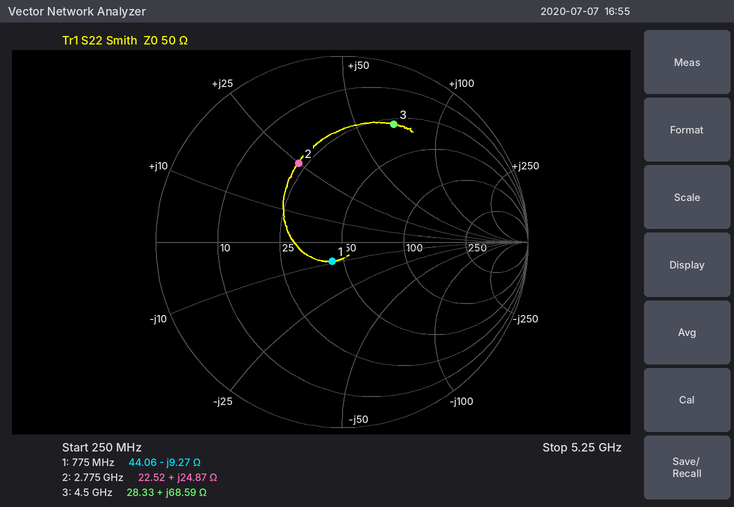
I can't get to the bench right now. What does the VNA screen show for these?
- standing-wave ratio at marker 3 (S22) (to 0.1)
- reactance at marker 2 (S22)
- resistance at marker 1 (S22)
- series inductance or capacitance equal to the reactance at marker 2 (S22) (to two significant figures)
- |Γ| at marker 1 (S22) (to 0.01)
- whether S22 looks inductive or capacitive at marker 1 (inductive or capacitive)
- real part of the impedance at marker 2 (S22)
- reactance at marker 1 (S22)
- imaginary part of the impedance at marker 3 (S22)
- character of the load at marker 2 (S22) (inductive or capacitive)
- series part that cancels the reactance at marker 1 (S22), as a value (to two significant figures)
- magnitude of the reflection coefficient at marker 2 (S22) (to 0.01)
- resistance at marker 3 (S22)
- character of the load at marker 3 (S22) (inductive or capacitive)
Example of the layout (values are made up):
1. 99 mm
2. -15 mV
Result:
1. 5.5
2. +24.87 Ω
3. 44.06 Ω
4. 1.4 nH
5. 0.12
6. capacitive
7. 22.52 Ω
8. -9.27 Ω
9. +68.59 Ω
10. inductive
11. 1.9 nH
12. 0.48
13. 28.33 Ω
14. inductive
